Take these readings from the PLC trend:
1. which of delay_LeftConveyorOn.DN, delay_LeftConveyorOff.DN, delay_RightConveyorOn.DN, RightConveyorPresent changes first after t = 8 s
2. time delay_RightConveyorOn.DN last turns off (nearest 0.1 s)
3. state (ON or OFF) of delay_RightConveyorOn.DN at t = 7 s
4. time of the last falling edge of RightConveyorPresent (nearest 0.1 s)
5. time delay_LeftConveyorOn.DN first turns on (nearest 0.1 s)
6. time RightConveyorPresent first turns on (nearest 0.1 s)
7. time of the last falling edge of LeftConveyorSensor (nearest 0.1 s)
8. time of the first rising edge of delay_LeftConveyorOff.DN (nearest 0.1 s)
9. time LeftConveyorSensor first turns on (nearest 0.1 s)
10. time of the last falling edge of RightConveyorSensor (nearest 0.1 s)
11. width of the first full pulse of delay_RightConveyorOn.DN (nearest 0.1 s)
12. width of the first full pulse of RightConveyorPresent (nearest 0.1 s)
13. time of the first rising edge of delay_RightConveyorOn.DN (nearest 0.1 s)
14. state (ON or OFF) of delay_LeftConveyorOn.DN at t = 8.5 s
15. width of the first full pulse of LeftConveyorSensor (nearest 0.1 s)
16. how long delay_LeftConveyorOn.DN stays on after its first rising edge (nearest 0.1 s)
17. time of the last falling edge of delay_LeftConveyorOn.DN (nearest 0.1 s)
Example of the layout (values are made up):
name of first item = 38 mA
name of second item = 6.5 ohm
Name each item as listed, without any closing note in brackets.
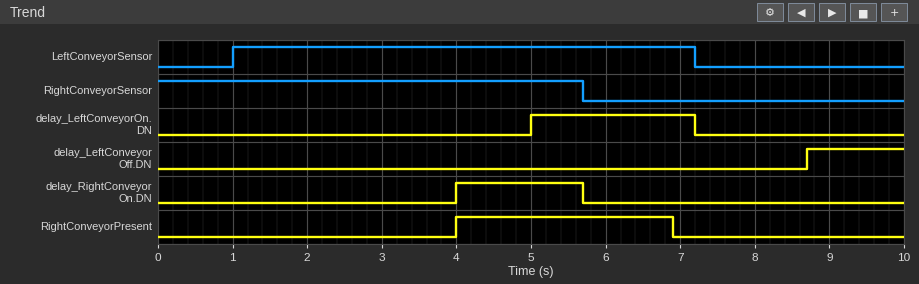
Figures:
which of delay_LeftConveyorOn.DN, delay_LeftConveyorOff.DN, delay_RightConveyorOn.DN, RightConveyorPresent changes first after t = 8 s = delay_LeftConveyorOff.DN
time delay_RightConveyorOn.DN last turns off = 5.7 s
state (ON or OFF) of delay_RightConveyorOn.DN at t = 7 s = OFF
time of the last falling edge of RightConveyorPresent = 6.9 s
time delay_LeftConveyorOn.DN first turns on = 5.0 s
time RightConveyorPresent first turns on = 4.0 s
time of the last falling edge of LeftConveyorSensor = 7.2 s
time of the first rising edge of delay_LeftConveyorOff.DN = 8.7 s
time LeftConveyorSensor first turns on = 1.0 s
time of the last falling edge of RightConveyorSensor = 5.7 s
width of the first full pulse of delay_RightConveyorOn.DN = 1.7 s
width of the first full pulse of RightConveyorPresent = 2.9 s
time of the first rising edge of delay_RightConveyorOn.DN = 4.0 s
state (ON or OFF) of delay_LeftConveyorOn.DN at t = 8.5 s = OFF
width of the first full pulse of LeftConveyorSensor = 6.2 s
how long delay_LeftConveyorOn.DN stays on after its first rising edge = 2.2 s
time of the last falling edge of delay_LeftConveyorOn.DN = 7.2 s
